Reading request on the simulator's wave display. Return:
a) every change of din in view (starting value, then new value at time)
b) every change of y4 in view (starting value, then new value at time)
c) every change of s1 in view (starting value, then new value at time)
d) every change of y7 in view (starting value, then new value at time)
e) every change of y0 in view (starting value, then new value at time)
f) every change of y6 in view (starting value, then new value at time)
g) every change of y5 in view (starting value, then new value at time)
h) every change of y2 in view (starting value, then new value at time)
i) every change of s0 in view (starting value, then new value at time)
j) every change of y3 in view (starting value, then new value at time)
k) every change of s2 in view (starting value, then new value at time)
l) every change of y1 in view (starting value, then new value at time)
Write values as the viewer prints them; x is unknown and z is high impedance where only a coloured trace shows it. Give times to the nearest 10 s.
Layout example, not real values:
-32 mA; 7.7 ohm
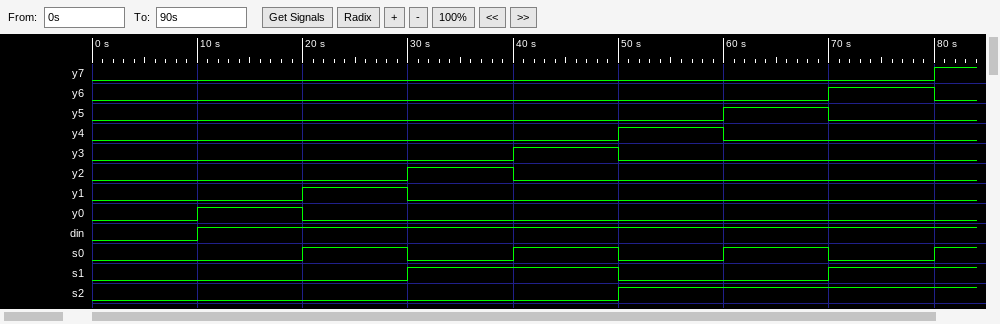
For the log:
0, 1 at 10 s; 0, 1 at 50 s, 0 at 60 s; 0, 1 at 30 s, 0 at 50 s, 1 at 70 s; 0, 1 at 80 s; 0, 1 at 10 s, 0 at 20 s; 0, 1 at 70 s, 0 at 80 s; 0, 1 at 60 s, 0 at 70 s; 0, 1 at 30 s, 0 at 40 s; 0, 1 at 20 s, 0 at 30 s, 1 at 40 s, 0 at 50 s, 1 at 60 s, 0 at 70 s, 1 at 80 s; 0, 1 at 40 s, 0 at 50 s; 0, 1 at 50 s; 0, 1 at 20 s, 0 at 30 s
